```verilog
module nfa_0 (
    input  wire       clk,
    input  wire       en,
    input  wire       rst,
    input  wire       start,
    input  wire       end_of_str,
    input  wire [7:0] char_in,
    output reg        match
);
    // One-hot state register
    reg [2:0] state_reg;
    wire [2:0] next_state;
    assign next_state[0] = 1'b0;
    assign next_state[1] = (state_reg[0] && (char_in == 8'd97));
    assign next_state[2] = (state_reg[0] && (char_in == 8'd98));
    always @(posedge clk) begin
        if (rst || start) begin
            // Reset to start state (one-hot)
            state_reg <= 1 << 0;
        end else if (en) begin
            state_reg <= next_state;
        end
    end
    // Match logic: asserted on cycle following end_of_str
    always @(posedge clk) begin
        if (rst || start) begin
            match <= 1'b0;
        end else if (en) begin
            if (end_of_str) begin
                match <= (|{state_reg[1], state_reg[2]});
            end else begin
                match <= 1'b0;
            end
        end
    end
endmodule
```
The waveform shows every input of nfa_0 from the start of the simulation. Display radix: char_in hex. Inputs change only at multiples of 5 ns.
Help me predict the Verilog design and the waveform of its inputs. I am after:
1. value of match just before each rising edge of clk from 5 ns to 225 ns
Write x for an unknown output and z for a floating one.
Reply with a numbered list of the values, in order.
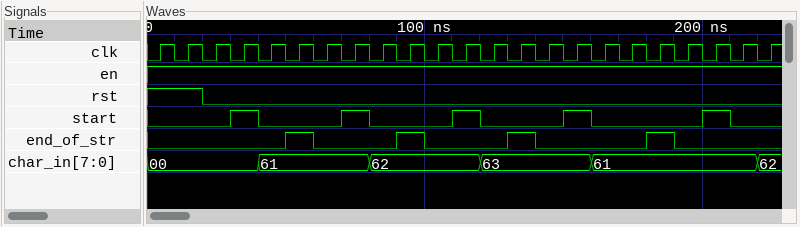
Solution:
1. x 0 0 0 0 0 1 0 0 0 1 0 0 0 0 0 0 0 0 0 0 0 0
